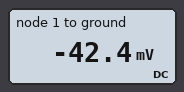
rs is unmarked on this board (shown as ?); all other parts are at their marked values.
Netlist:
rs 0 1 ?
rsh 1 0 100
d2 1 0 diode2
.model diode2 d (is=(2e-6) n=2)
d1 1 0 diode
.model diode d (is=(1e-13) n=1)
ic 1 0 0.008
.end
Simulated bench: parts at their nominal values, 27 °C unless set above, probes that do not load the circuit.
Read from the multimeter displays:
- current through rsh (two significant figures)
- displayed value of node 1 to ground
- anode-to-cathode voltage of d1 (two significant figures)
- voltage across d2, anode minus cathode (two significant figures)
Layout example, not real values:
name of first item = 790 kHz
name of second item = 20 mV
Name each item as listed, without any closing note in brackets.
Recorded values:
current through rsh = 420 µA
displayed value of node 1 to ground = -42.4 mV
anode-to-cathode voltage of d1 = -42 mV
voltage across d2, anode minus cathode = -42 mV
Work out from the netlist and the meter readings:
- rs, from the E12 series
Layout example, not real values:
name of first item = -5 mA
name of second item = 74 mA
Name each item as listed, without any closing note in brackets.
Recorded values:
rs, from the E12 series = 5.6 Ω
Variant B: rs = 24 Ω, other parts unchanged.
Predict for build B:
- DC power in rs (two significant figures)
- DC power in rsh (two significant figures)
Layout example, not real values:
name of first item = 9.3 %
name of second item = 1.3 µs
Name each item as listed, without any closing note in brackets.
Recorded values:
DC power in rs = 1.0 mW
DC power in rsh = 240 µW
